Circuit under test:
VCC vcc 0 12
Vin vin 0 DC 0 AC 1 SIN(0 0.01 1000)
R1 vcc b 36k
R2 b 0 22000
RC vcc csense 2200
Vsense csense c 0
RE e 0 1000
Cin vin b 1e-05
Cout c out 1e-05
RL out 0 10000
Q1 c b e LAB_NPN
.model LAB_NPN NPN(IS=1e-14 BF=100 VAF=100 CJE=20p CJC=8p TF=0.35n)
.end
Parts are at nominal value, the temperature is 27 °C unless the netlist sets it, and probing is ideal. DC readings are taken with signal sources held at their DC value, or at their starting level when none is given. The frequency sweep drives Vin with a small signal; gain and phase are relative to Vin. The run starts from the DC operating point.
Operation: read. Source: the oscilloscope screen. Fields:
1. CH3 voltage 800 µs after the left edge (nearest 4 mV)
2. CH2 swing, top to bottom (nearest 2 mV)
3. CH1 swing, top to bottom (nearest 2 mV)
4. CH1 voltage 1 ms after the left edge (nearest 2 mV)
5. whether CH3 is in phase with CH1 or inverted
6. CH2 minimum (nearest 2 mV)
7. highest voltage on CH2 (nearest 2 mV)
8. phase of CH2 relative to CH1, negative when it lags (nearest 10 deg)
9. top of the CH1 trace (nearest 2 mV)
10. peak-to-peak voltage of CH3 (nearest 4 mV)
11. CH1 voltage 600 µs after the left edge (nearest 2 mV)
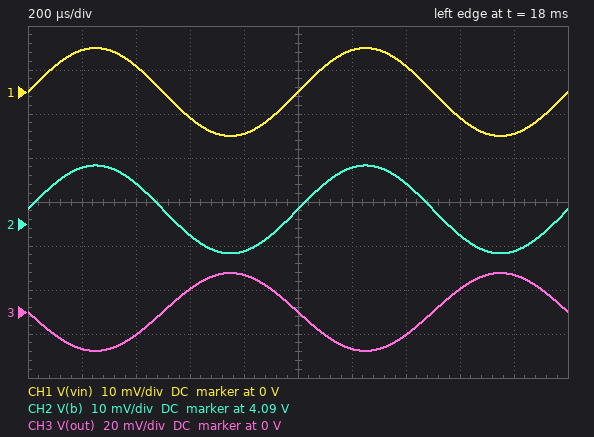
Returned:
16 mV
20 mV
20 mV
0 V
inverted
4.084 V
4.104 V
0 deg
10 mV
36 mV
-6 mV
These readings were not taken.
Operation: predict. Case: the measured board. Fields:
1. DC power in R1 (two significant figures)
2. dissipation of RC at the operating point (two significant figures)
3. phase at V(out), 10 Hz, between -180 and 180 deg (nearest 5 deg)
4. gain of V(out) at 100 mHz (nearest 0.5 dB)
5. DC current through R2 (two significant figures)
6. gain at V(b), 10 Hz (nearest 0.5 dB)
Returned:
1.7 mW
25 mW
-165 deg
-40.0 dB
190 µA
0 dB
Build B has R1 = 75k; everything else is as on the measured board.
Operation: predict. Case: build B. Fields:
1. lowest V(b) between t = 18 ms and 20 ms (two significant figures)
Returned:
2.4 V
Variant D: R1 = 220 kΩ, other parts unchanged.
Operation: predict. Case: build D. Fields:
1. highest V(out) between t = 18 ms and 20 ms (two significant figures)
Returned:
17 mV
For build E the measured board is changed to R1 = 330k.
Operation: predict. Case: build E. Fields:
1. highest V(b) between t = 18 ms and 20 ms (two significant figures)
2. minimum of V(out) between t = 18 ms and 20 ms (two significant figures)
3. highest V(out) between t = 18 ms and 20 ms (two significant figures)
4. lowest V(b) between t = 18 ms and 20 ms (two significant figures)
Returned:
740 mV
-15 mV
15 mV
720 mV
